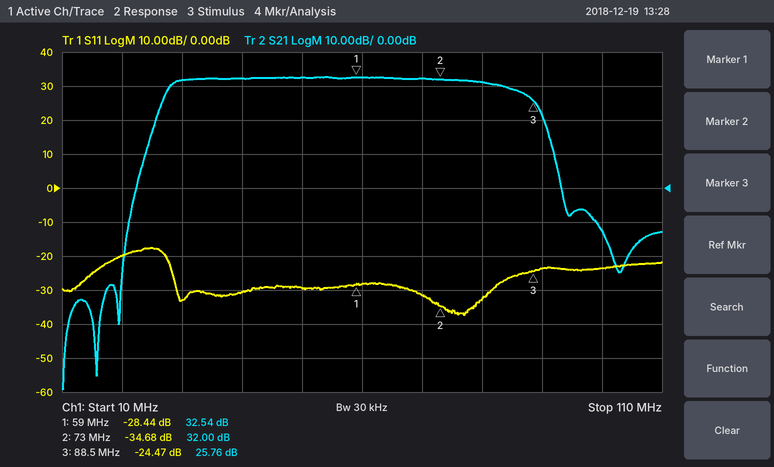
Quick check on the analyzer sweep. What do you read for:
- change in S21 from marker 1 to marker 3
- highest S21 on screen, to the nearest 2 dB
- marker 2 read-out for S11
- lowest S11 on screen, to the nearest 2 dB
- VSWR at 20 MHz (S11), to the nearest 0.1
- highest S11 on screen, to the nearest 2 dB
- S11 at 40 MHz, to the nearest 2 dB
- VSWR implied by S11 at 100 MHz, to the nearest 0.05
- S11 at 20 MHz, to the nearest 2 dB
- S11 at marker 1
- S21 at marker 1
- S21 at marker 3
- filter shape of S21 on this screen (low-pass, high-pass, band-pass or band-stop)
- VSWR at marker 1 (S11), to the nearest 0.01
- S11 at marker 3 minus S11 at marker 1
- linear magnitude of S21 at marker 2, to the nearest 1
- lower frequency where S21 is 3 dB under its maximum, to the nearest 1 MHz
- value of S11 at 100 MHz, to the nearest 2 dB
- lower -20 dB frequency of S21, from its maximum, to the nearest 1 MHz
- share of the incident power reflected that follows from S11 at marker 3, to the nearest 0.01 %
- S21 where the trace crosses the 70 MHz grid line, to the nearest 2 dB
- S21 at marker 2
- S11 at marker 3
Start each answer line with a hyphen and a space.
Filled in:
- -6.78 dB
- 32 dB
- -34.68 dB
- -38 dB
- 1.2
- -18 dB
- -30 dB
- 1.15
- -20 dB
- -28.44 dB
- 32.54 dB
- 25.76 dB
- band-pass
- 1.08
- 3.97 dB
- 40
- 28 MHz
- -24 dB
- 24 MHz
- 0.36 %
- 32 dB
- 32.00 dB
- -24.47 dB
